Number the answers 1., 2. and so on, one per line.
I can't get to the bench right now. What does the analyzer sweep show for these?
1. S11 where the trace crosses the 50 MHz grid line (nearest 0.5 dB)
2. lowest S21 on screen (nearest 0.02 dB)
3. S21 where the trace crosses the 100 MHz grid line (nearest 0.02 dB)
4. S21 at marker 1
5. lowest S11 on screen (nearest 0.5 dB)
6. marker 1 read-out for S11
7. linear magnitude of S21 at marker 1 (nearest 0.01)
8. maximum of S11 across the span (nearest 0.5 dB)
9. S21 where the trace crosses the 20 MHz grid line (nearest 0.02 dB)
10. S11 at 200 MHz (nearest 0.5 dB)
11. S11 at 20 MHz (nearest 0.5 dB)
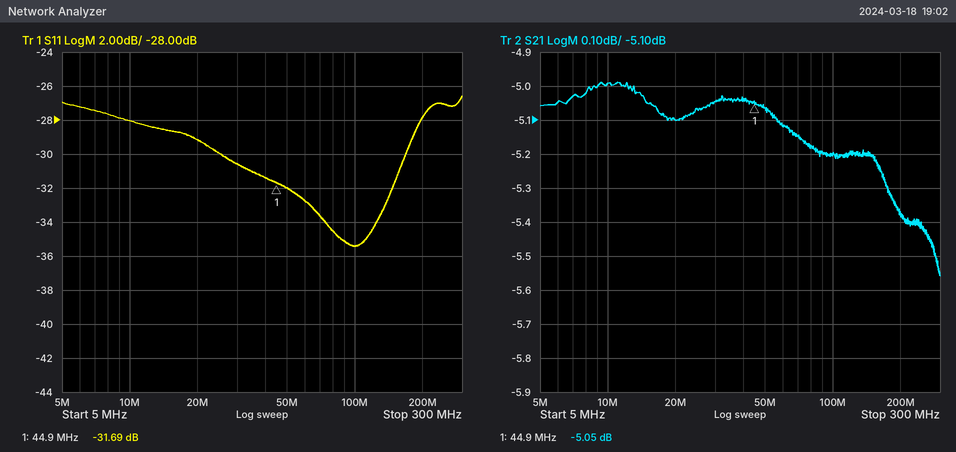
1. -32.0 dB
2. -5.56 dB
3. -5.20 dB
4. -5.05 dB
5. -35.5 dB
6. -31.69 dB
7. 0.56
8. -26.5 dB
9. -5.10 dB
10. -28.0 dB
11. -29.0 dB
